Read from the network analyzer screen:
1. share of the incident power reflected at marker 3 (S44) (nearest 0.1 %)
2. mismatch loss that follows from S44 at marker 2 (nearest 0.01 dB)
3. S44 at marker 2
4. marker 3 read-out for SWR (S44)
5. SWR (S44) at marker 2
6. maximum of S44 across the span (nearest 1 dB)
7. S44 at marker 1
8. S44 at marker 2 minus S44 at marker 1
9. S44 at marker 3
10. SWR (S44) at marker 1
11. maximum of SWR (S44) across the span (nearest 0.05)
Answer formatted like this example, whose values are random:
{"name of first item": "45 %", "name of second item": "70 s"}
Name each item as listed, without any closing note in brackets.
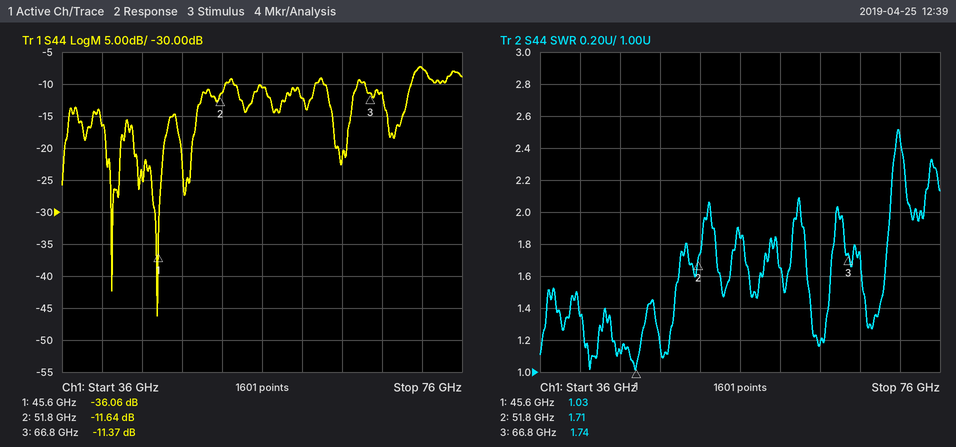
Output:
{"share of the incident power reflected at marker 3 (S44)": "7.3 %", "mismatch loss that follows from S44 at marker 2": "0.31 dB", "S44 at marker 2": "-11.64 dB", "marker 3 read-out for SWR": "1.74", "SWR (S44) at marker 2": "1.71", "maximum of S44 across the span": "-7 dB", "S44 at marker 1": "-36.06 dB", "S44 at marker 2 minus S44 at marker 1": "24.42 dB", "S44 at marker 3": "-11.37 dB", "SWR (S44) at marker 1": "1.03", "maximum of SWR (S44) across the span": "2.50"}
